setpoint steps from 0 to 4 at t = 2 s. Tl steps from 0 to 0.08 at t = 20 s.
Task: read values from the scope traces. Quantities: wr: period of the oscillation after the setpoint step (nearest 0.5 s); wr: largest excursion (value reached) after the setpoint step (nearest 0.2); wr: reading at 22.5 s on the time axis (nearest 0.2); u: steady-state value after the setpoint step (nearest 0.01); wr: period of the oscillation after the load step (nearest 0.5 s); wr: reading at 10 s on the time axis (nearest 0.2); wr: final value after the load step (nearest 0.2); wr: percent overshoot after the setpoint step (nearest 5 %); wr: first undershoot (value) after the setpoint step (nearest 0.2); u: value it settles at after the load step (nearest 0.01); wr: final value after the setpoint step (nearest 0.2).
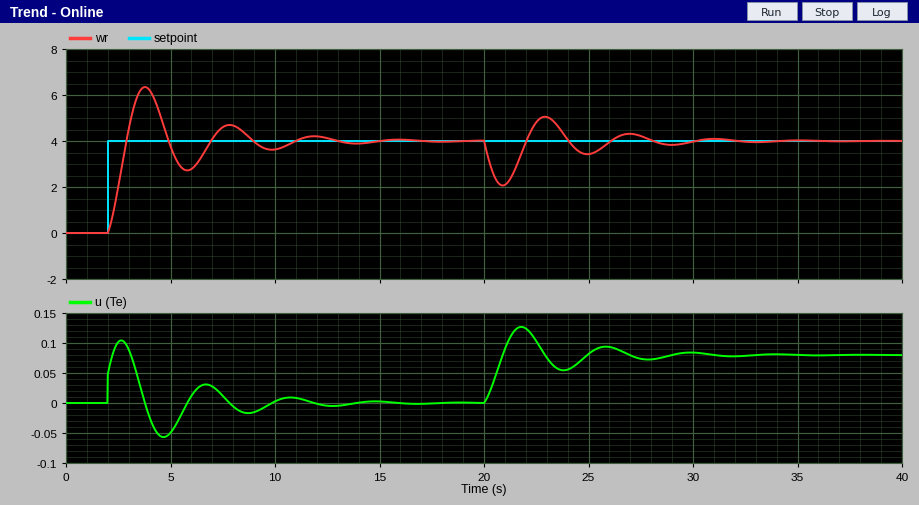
4.0 s
6.4
4.8
0.00
4.0 s
3.6
4.0
60 %
2.8
0.08
4.0
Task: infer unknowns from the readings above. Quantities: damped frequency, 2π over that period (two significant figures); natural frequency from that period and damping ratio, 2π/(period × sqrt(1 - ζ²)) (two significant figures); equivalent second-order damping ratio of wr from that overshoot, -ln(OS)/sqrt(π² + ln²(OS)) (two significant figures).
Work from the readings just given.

1.6 rad/s
1.6 rad/s
0.16
